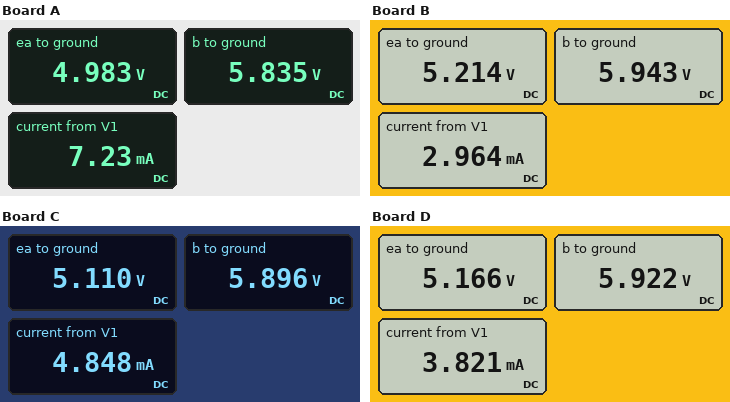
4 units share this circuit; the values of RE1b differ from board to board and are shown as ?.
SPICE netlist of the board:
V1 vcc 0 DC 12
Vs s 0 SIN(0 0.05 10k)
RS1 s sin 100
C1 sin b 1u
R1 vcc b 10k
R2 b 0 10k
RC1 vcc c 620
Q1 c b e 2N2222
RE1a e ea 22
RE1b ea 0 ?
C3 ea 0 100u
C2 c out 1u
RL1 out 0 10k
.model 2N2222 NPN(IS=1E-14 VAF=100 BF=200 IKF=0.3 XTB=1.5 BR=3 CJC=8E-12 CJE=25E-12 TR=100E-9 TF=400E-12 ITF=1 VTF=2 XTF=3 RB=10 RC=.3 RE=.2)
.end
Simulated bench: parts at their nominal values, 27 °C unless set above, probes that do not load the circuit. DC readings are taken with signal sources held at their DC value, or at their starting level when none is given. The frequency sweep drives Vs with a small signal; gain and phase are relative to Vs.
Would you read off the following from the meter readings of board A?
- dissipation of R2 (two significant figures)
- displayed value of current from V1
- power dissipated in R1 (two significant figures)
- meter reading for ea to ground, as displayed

3.4 mW
7.23 mA
3.8 mW
4.983 V
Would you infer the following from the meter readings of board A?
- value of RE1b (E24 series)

750 Ω
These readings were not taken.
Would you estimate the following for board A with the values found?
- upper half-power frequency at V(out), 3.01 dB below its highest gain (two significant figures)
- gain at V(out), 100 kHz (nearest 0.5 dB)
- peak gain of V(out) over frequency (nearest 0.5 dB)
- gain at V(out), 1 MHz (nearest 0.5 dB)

8.9 MHz
26.5 dB
26.5 dB
26.5 dB
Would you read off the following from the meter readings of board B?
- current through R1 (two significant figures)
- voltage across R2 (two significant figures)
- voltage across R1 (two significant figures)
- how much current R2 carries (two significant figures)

610 µA
5.9 V
6.1 V
590 µA
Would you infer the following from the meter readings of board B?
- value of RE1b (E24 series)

2.2 kΩ
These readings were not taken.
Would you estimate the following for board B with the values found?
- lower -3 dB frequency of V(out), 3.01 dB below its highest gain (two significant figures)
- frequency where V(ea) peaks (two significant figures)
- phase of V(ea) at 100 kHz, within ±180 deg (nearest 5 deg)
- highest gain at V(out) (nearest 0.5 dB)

89 Hz
39 Hz
-90 deg
24.5 dB
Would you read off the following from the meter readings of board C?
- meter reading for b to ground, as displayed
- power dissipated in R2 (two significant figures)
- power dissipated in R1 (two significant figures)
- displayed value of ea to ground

5.896 V
3.5 mW
3.7 mW
5.110 V
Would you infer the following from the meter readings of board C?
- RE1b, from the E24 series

1.2 kΩ
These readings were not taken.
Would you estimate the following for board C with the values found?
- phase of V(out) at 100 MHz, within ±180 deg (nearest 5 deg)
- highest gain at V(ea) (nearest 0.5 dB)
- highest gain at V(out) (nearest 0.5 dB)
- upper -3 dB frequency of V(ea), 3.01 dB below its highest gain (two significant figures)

75 deg
-6.5 dB
26.0 dB
130 Hz
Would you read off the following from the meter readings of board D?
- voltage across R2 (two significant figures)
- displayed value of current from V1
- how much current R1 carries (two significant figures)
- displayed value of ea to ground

5.9 V
3.821 mA
610 µA
5.166 V
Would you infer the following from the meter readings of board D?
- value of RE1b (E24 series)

1.6 kΩ
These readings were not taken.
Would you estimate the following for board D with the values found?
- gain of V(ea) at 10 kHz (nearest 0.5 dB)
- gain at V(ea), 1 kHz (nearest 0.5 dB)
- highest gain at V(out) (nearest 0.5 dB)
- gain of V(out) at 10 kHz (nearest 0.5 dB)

-46.0 dB
-26.0 dB
25.5 dB
25.5 dB
